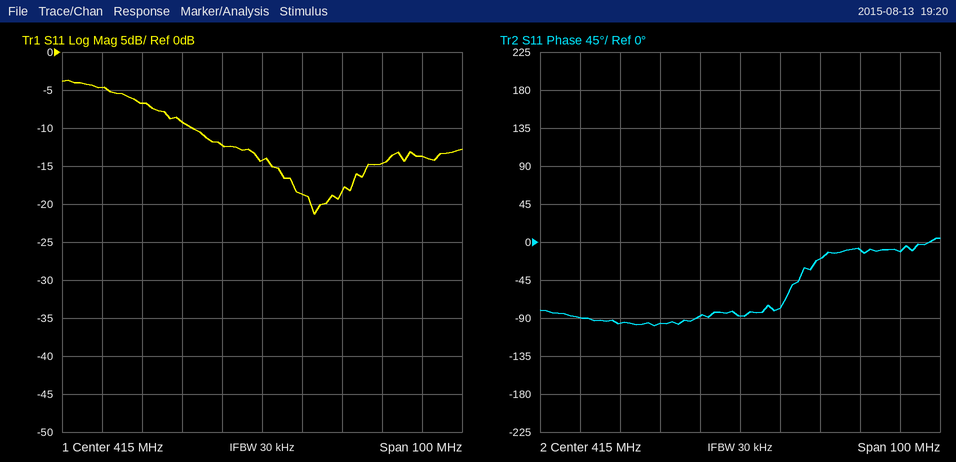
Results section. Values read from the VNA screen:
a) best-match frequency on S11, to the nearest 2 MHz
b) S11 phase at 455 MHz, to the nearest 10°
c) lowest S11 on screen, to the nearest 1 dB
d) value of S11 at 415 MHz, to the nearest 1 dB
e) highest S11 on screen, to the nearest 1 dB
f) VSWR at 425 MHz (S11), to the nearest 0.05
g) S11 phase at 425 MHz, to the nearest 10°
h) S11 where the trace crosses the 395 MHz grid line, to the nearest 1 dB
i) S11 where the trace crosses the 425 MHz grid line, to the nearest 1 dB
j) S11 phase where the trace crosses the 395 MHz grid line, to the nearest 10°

428 MHz
-10°
-21 dB
-14 dB
-4 dB
1.25
-80°
-9 dB
-19 dB
-100°
